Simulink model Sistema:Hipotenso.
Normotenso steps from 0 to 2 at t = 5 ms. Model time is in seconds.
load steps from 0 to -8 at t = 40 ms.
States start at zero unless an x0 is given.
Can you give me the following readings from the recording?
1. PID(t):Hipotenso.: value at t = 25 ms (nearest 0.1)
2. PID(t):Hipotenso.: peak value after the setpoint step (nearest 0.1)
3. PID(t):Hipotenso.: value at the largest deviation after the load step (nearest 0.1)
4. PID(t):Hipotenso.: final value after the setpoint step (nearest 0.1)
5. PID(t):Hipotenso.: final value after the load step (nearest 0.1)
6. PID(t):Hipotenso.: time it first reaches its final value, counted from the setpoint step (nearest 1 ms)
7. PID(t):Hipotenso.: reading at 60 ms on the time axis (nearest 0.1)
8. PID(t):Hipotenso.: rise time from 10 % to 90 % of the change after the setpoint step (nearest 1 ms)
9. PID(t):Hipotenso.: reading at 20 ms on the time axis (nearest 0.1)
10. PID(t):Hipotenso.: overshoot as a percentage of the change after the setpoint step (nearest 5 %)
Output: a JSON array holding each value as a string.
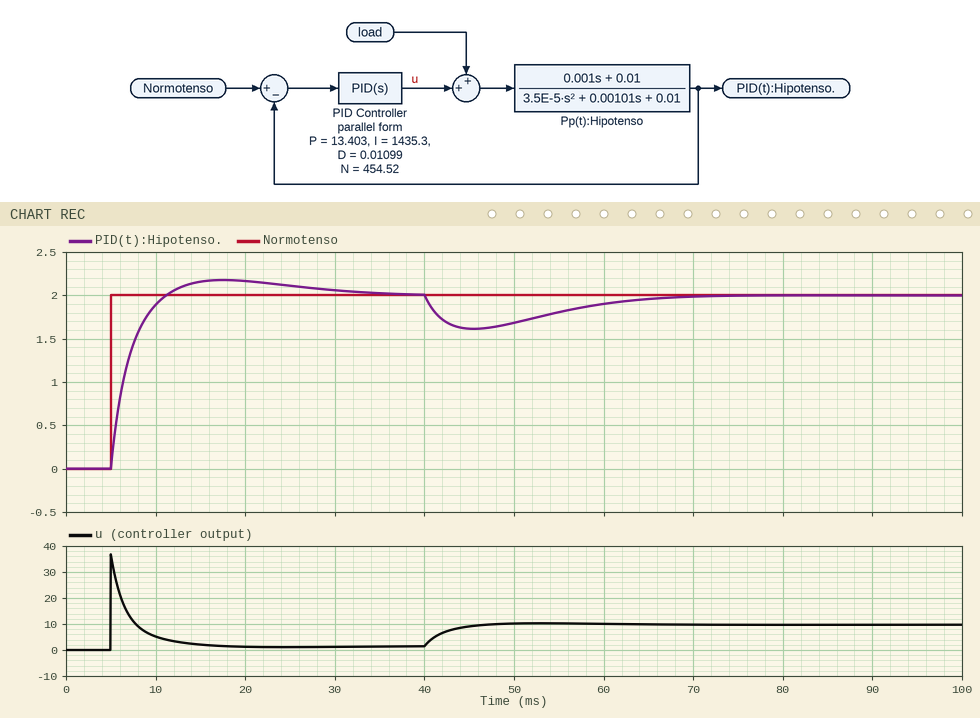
["2.1", "2.2", "1.6", "2.0", "2.0", "6 ms", "1.9", "4 ms", "2.2", "10 %"]
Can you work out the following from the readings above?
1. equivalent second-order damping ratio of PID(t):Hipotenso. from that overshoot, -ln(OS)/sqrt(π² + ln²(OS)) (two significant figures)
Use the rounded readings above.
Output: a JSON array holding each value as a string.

["0.59"]
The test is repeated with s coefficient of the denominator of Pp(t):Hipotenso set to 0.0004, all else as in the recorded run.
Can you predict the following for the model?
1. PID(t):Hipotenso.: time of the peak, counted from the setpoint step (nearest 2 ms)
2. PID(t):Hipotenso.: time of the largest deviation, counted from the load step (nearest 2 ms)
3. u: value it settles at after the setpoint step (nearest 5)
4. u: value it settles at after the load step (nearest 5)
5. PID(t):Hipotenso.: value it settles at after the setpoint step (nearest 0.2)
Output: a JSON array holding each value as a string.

["12 ms", "6 ms", "0", "10", "2.0"]
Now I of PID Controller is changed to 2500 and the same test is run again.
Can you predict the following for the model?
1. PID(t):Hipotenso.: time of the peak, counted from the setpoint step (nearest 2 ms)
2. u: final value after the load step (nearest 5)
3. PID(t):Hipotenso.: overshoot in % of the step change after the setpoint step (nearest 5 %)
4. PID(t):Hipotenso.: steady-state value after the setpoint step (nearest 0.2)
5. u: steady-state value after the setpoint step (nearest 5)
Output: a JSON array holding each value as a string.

["10 ms", "10", "15 %", "2.0", "0"]
